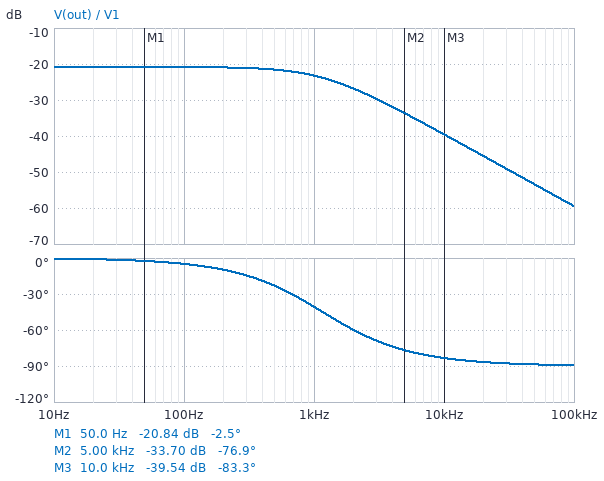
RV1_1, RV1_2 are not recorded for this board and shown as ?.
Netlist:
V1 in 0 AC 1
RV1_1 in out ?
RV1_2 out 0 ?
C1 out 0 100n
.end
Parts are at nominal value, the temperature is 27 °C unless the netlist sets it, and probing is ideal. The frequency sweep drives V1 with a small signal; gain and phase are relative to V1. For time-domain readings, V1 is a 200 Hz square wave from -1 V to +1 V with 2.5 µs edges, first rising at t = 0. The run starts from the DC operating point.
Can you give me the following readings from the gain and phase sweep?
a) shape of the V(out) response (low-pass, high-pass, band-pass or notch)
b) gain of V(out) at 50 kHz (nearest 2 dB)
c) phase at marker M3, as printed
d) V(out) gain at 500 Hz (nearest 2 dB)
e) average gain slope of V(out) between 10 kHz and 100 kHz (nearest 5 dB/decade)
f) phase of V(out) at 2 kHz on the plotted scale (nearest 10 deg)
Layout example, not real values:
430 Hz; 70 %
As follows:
low-pass; -54 dB; -83.3 deg; -22 dB; -20 dB/decade; -60 deg
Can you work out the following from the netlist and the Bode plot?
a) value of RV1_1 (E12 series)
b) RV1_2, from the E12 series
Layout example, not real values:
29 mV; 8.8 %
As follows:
15 kΩ; 1.5 kΩ
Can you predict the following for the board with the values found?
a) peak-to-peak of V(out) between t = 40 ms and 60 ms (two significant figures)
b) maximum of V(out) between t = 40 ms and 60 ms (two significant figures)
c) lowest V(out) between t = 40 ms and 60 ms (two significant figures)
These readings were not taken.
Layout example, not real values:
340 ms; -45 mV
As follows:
180 mV; 91 mV; -91 mV
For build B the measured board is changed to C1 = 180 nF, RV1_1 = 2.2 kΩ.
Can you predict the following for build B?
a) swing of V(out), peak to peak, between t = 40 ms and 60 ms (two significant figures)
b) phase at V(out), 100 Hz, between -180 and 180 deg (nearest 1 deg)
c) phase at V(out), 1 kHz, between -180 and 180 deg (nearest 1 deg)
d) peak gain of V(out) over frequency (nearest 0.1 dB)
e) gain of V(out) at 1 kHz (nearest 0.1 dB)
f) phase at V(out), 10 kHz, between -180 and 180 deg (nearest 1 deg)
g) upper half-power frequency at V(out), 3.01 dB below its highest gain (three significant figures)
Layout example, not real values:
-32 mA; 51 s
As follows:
810 mV; -6 deg; -45 deg; -7.8 dB; -10.9 dB; -84 deg; 991 Hz
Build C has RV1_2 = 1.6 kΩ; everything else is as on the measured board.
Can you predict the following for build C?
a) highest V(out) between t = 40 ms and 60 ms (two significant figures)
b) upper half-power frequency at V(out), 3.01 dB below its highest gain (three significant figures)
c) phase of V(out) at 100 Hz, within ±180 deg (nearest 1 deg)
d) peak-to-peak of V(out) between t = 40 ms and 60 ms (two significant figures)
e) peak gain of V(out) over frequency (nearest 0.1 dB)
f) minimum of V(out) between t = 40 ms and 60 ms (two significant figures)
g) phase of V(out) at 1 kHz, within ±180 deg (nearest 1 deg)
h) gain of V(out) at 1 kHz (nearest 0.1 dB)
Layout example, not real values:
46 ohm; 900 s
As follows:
96 mV; 1.10 kHz; -5 deg; 190 mV; -20.3 dB; -96 mV; -42 deg; -22.9 dB
